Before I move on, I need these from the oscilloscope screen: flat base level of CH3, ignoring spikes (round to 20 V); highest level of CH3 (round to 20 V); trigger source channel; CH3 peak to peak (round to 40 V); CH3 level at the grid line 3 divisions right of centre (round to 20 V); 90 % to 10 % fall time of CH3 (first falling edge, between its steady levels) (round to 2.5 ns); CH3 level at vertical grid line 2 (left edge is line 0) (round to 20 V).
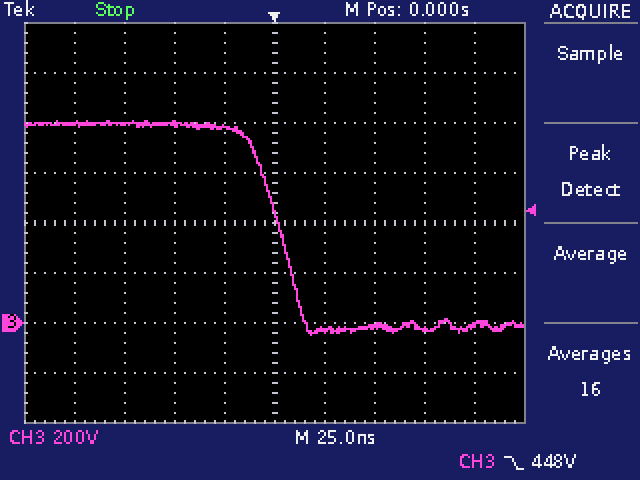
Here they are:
-20 V
800 V
CH3
840 V
-20 V
25.0 ns
800 V
